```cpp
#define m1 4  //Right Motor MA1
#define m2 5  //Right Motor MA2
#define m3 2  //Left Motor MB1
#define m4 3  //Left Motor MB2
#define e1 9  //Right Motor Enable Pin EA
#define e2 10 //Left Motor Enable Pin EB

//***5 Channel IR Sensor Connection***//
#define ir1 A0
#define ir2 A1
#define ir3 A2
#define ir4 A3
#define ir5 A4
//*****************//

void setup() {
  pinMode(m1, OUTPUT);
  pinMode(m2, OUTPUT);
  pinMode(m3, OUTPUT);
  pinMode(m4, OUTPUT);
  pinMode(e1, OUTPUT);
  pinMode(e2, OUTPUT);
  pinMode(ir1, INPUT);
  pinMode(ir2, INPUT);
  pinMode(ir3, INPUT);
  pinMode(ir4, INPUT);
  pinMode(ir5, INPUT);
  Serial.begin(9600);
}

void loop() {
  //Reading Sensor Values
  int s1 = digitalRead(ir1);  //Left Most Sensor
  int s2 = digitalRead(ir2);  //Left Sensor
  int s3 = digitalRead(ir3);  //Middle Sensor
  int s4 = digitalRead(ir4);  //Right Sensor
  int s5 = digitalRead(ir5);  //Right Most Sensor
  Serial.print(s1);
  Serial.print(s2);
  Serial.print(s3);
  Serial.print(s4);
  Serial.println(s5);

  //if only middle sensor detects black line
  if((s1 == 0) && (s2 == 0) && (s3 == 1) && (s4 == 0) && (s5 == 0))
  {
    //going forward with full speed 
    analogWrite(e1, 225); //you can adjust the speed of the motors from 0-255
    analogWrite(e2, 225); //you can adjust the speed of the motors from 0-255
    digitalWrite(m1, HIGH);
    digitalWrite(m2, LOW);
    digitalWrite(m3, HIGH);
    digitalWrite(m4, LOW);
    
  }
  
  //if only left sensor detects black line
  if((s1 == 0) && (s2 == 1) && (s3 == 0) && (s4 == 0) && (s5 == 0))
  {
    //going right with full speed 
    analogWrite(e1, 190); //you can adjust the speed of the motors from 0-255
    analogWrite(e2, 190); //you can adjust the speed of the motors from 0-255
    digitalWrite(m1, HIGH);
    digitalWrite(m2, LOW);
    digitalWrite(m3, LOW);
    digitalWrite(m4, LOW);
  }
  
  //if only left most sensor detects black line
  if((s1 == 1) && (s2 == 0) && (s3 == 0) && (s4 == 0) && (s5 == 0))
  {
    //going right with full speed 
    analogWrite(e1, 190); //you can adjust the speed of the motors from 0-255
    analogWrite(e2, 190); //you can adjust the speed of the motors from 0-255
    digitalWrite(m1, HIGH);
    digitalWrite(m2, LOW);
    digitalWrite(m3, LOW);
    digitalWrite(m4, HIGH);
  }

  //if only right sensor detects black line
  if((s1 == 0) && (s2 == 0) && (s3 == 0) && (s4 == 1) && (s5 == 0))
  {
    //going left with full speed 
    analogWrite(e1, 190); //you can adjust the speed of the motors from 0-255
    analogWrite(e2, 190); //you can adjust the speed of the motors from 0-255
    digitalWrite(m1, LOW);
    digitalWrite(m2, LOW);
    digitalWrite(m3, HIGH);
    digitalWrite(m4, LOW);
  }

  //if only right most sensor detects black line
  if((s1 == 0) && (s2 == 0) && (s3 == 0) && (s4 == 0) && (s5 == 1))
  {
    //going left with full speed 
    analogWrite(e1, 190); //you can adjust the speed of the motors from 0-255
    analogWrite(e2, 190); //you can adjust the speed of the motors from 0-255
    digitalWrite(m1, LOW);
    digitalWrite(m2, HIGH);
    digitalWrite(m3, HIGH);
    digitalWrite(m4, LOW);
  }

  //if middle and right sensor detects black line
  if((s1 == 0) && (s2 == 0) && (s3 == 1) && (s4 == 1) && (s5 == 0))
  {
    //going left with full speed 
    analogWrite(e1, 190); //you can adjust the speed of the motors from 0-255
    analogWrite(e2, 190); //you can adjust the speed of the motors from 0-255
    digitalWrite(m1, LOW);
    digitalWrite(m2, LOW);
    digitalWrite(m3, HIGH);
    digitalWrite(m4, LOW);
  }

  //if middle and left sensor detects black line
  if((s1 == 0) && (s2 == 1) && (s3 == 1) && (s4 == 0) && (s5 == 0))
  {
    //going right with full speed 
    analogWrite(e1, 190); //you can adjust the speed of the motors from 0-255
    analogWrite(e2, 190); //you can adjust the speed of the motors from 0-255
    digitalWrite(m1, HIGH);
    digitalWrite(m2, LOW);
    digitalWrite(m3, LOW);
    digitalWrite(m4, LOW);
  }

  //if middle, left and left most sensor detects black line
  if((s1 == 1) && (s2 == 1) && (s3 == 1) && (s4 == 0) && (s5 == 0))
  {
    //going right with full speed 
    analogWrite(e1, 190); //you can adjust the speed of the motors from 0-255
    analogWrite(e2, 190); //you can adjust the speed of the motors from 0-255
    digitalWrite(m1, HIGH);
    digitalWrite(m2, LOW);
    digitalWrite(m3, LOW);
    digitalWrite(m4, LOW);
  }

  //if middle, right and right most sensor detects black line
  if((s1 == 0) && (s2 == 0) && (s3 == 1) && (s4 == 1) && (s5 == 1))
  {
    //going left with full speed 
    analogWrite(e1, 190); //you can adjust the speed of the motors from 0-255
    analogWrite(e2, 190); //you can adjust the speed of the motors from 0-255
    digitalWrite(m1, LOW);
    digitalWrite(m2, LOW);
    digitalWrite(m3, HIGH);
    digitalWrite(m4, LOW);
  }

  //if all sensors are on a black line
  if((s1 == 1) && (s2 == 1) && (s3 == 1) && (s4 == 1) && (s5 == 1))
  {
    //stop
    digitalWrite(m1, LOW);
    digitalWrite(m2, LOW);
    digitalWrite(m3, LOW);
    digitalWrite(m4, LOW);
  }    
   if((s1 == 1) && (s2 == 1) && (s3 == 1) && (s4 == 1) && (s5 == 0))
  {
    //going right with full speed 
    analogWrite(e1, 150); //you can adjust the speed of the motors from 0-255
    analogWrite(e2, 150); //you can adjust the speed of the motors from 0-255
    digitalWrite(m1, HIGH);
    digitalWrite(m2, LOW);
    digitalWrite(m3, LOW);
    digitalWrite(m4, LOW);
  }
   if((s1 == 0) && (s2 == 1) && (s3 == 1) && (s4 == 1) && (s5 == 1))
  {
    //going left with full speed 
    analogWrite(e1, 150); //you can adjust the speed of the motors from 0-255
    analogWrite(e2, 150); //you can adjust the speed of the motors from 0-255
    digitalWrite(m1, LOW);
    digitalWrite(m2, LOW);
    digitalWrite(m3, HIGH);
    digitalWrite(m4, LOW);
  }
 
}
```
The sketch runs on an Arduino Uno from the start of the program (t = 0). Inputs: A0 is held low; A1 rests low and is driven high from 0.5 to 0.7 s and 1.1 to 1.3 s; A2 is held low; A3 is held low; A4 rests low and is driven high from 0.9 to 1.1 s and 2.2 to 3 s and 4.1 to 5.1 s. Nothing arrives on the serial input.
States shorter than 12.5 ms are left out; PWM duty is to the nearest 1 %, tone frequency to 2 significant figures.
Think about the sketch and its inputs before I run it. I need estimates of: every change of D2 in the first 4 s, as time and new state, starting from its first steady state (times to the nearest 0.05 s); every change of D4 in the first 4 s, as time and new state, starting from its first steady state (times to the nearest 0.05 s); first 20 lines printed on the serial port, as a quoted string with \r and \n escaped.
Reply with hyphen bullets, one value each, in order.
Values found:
- 0 s low; 0.9 s high; 1.1 s low; 2.2 s high
- 0 s low; 0.5 s high; 0.9 s low; 1.1 s high; 2.2 s low
- "00000\r\n00000\r\n00000\r\n00000\r\n00000\r\n00000\r\n00000\r\n00000\r\n00000\r\n00000\r\n00000\r\n00000\r\n00000\r\n00000\r\n00000\r\n00000\r\n00000\r\n00000\r\n00000\r\n00000\r\n"
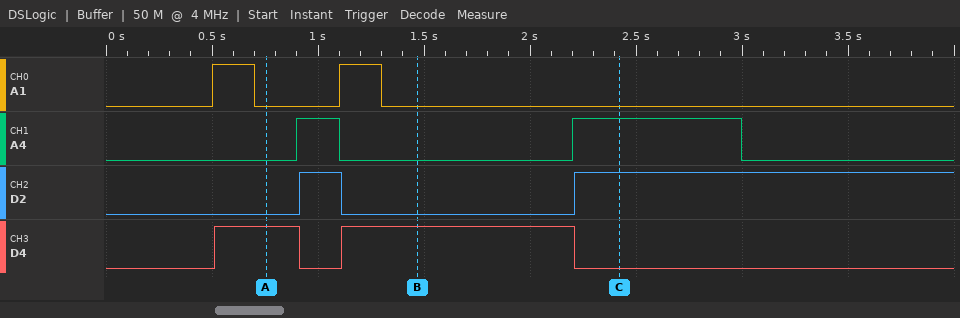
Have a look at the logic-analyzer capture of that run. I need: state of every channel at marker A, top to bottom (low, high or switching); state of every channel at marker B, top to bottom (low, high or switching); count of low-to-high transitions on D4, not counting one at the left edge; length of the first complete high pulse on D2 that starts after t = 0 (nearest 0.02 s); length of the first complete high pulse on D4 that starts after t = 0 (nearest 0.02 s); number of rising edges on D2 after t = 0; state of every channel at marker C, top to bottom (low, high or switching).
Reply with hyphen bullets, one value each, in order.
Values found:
- A1 low, A4 low, D2 low, D4 high
- A1 low, A4 low, D2 low, D4 high
- 2
- 0.20 s
- 0.40 s
- 2
- A1 low, A4 high, D2 high, D4 low
